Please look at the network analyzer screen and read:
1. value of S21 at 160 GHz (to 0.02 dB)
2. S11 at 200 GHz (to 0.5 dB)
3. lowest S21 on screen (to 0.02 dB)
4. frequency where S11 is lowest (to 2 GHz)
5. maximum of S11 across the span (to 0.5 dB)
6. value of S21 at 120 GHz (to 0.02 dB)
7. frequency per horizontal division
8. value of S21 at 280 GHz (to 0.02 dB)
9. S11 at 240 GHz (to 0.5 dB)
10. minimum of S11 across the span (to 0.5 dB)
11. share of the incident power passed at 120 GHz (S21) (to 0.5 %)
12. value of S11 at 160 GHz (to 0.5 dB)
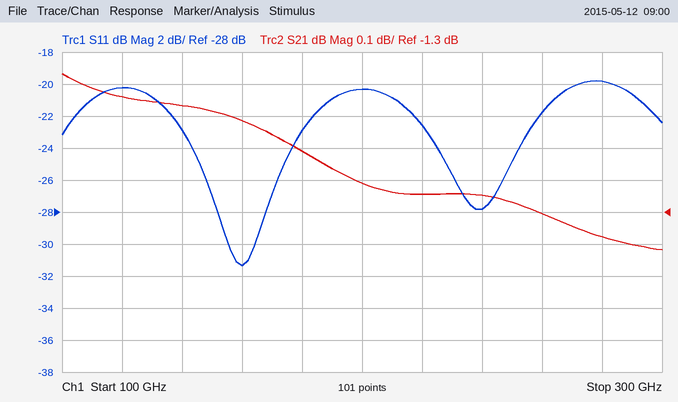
-1.02 dB
-20.5 dB
-1.42 dB
160 GHz
-20.0 dB
-0.94 dB
20 GHz
-1.38 dB
-28.0 dB
-31.5 dB
80.5 %
-31.5 dB
